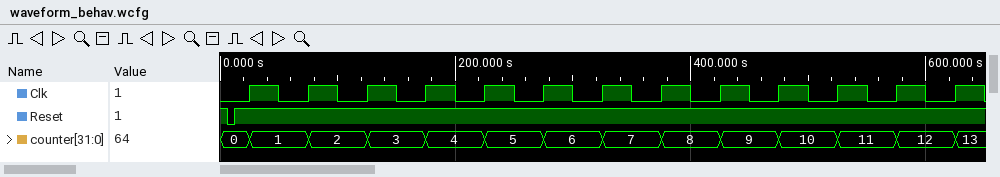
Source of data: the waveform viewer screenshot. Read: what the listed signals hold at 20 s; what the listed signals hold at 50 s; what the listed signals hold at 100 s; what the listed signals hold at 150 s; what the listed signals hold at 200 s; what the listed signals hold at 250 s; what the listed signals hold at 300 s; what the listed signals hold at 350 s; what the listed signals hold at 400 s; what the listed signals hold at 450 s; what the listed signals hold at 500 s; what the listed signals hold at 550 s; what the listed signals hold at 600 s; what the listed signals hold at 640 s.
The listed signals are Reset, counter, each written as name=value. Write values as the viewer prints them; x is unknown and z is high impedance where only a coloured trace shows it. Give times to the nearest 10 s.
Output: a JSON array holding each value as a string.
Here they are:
["Reset=1, counter=0", "Reset=1, counter=1", "Reset=1, counter=2", "Reset=1, counter=3", "Reset=1, counter=4", "Reset=1, counter=5", "Reset=1, counter=6", "Reset=1, counter=7", "Reset=1, counter=8", "Reset=1, counter=9", "Reset=1, counter=10", "Reset=1, counter=11", "Reset=1, counter=12", "Reset=1, counter=13"]
